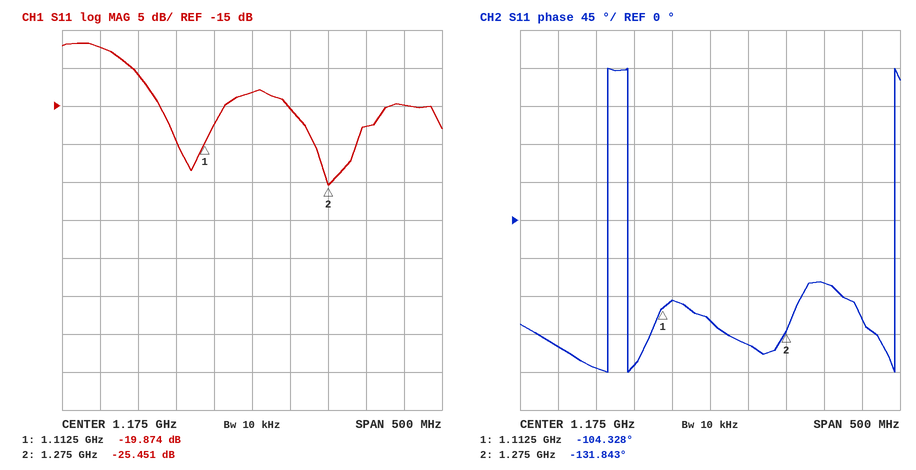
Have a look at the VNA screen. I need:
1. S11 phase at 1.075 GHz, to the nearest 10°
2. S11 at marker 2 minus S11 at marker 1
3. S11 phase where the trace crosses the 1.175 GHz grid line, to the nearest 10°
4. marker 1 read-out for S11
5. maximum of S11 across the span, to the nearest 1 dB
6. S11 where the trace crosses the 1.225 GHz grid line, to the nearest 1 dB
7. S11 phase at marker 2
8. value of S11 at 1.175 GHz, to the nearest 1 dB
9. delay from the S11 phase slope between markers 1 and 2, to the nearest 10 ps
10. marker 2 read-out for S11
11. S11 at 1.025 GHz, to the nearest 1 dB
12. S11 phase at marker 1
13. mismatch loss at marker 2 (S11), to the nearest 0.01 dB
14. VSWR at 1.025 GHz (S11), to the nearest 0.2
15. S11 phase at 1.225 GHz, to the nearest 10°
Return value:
-170°
-5.577 dB
-120°
-19.874 dB
-7 dB
-15 dB
-131.843°
-13 dB
470 ps
-25.451 dB
-11 dB
-104.328°
0.01 dB
1.8
-150°
